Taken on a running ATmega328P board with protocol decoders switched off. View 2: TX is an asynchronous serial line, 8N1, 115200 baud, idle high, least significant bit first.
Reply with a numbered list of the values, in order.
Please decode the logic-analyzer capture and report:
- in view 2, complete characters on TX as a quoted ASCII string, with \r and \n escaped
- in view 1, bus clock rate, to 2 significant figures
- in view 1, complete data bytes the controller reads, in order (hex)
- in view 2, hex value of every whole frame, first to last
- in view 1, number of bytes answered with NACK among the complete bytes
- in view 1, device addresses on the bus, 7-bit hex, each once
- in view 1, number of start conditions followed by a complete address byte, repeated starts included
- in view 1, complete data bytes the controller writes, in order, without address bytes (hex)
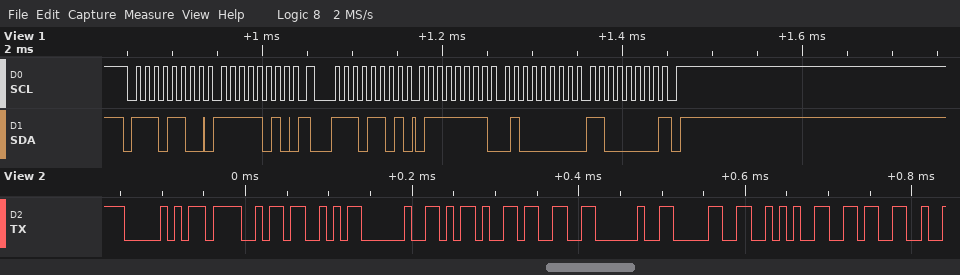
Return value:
1. "POS -3 0*6"
2. 100 kHz
3. 7F 40 C0
4. 50 4F 53 20 2D 33 20 30 2A 36
5. 1
6. 0x76
7. 2
8. FA
